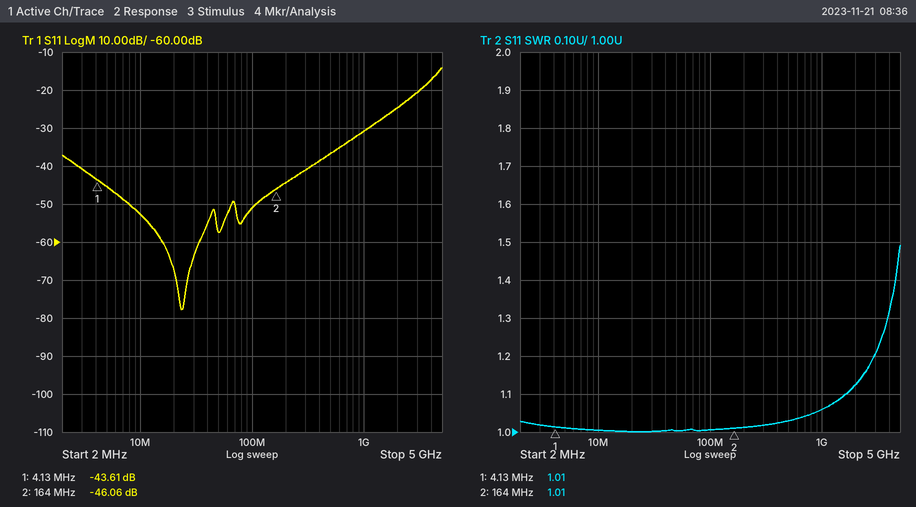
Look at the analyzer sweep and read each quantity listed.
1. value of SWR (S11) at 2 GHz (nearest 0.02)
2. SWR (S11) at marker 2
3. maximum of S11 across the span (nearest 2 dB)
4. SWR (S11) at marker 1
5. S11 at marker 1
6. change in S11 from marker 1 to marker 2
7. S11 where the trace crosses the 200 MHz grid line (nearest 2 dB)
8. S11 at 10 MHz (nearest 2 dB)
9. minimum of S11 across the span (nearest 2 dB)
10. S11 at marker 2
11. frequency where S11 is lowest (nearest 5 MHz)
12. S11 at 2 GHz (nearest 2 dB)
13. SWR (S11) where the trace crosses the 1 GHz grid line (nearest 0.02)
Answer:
1.12
1.01
-14 dB
1.01
-43.61 dB
-2.45 dB
-44 dB
-52 dB
-78 dB
-46.06 dB
25 MHz
-24 dB
1.06
